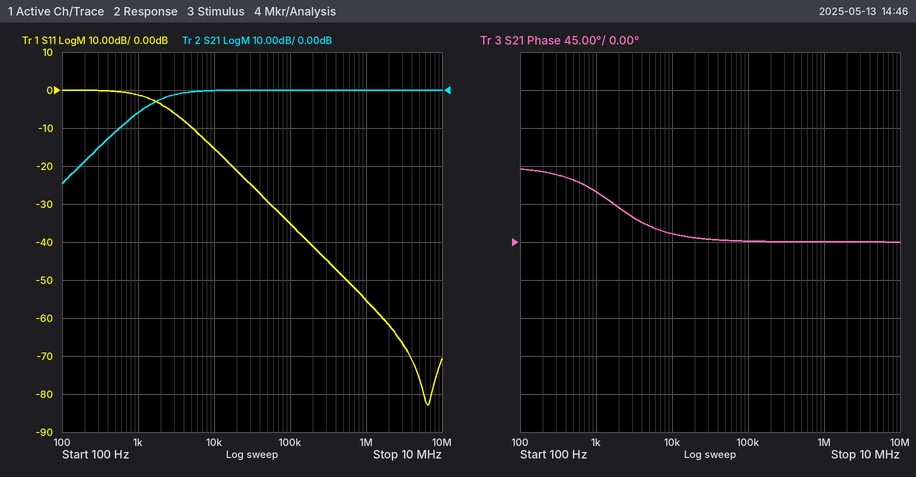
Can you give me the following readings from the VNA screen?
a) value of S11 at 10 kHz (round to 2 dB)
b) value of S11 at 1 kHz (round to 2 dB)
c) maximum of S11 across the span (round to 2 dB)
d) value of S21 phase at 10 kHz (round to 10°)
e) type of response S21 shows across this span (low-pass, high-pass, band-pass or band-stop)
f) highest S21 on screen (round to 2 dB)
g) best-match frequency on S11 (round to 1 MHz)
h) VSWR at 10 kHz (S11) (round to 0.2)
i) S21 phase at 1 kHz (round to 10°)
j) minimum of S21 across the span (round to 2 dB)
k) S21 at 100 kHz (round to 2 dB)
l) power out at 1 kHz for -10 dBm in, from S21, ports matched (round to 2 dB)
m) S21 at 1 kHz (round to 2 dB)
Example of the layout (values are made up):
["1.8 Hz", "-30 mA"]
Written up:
["-16 dB", "-2 dB", "0 dB", "10°", "high-pass", "0 dB", "6 MHz", "1.4", "60°", "-24 dB", "0 dB", "-16 dBm", "-6 dB"]
